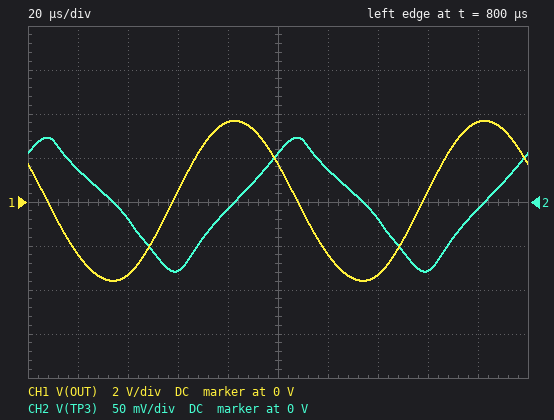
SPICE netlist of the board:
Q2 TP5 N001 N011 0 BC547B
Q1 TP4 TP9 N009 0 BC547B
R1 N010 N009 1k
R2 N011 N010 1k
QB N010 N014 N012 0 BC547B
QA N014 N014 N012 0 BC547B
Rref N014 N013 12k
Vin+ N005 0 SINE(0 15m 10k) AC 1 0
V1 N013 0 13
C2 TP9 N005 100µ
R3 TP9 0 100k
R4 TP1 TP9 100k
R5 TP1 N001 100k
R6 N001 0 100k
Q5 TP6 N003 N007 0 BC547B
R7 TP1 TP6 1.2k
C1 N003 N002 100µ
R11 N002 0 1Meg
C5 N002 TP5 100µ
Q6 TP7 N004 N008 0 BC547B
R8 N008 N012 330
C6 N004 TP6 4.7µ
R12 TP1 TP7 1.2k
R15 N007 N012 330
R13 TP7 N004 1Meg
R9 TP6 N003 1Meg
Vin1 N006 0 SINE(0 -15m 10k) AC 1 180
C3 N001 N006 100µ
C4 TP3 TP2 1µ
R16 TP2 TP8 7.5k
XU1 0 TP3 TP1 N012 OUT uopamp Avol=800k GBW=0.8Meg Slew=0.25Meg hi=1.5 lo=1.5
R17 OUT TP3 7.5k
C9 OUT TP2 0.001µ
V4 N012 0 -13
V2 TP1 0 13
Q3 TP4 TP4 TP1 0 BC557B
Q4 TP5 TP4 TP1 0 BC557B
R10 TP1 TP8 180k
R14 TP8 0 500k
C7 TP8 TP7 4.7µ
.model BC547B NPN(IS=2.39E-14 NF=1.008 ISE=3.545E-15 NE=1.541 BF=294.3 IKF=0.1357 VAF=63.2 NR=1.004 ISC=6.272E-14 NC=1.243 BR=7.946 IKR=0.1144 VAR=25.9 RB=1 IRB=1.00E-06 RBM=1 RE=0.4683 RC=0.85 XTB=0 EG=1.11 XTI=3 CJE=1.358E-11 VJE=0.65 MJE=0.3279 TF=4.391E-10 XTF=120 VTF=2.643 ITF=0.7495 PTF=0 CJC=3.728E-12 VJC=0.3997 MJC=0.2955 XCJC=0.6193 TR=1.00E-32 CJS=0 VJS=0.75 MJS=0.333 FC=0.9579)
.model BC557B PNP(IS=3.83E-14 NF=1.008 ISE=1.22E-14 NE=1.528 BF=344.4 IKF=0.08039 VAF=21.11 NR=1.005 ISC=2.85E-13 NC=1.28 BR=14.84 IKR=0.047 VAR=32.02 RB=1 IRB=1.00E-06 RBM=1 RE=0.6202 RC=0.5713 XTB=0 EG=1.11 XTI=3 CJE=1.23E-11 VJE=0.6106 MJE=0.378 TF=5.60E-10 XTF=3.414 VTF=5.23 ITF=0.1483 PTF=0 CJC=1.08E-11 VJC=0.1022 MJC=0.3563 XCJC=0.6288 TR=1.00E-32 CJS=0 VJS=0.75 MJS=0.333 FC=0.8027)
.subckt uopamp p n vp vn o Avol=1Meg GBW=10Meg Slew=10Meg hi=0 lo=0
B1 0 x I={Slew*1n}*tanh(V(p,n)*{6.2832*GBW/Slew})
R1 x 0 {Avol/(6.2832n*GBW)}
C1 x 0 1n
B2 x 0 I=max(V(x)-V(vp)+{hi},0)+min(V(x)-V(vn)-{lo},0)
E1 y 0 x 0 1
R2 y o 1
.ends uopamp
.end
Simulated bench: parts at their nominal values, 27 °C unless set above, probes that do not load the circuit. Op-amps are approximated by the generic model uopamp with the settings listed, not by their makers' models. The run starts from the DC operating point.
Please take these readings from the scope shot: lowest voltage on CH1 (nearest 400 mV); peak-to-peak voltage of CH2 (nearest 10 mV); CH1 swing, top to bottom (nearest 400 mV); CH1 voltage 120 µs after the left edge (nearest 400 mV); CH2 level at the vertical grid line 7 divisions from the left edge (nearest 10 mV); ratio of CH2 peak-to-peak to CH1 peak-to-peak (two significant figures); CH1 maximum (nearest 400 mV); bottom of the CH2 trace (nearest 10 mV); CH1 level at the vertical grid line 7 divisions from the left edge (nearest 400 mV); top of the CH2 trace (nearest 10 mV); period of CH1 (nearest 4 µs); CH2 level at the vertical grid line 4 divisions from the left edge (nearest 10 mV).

-3.6 V
150 mV
7.2 V
-2.4 V
-20 mV
0.021
3.6 V
-80 mV
-3.2 V
70 mV
100 µs
-10 mV
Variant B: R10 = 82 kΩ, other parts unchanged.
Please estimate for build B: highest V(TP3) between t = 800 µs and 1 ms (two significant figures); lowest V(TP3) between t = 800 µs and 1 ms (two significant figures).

72 mV
-77 mV
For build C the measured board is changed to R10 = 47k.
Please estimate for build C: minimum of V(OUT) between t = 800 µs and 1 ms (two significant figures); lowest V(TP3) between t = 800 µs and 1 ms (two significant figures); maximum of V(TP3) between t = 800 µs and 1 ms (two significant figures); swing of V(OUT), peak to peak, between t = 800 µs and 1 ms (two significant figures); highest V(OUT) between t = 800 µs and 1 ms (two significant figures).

-3.5 V
-75 mV
70 mV
7.2 V
3.6 V
